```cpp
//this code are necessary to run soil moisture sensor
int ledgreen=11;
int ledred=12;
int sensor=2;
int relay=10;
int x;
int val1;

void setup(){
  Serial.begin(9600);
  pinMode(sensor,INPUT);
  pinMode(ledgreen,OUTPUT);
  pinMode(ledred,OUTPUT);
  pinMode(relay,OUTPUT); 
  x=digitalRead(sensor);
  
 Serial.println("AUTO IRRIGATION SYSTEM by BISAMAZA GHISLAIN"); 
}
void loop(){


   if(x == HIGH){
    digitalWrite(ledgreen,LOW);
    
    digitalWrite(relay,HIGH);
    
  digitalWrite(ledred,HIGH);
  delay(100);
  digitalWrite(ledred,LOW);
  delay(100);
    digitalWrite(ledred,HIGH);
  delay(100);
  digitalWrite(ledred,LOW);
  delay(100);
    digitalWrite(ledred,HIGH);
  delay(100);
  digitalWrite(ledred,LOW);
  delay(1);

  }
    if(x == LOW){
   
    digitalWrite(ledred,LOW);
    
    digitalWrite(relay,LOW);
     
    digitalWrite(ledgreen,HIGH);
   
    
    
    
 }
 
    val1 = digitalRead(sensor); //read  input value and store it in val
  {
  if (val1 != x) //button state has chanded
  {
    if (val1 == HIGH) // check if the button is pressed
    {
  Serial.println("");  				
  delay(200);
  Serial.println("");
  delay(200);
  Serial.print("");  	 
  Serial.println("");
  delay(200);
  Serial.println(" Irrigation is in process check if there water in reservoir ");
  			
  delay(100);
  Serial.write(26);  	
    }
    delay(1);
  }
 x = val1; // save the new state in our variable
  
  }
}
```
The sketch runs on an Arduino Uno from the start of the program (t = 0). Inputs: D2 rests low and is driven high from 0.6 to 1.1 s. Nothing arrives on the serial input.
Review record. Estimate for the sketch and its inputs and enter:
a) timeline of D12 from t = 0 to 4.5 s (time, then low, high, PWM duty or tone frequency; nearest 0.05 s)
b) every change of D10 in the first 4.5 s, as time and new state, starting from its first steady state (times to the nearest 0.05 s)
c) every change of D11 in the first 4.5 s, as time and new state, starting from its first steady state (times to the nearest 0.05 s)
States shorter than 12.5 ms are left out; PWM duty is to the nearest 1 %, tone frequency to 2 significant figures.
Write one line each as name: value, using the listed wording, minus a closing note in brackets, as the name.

timeline of D12 from t = 0 to 4.5 s: 0 s low; 1.3 s high; 1.4 s low; 1.5 s high; 1.6 s low; 1.7 s high; 1.8 s low
every change of D10 in the first 4.5 s, as time and new state, starting from its first steady state: 0 s low; 1.3 s high; 1.8 s low
every change of D11 in the first 4.5 s, as time and new state, starting from its first steady state: 0 s high; 1.3 s low; 1.8 s high
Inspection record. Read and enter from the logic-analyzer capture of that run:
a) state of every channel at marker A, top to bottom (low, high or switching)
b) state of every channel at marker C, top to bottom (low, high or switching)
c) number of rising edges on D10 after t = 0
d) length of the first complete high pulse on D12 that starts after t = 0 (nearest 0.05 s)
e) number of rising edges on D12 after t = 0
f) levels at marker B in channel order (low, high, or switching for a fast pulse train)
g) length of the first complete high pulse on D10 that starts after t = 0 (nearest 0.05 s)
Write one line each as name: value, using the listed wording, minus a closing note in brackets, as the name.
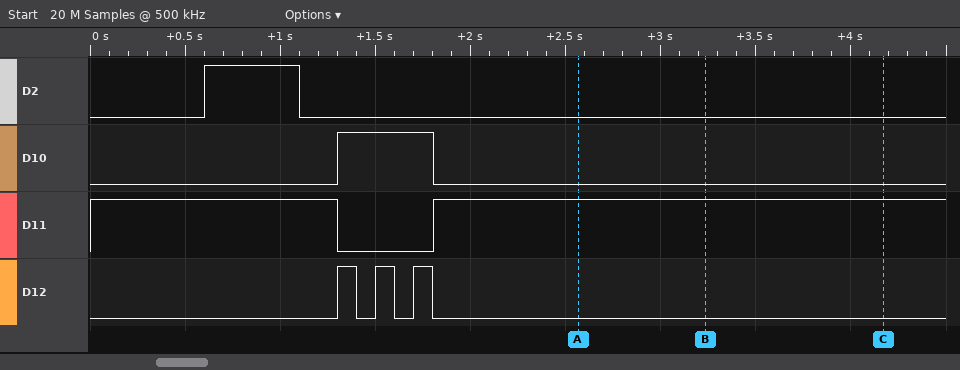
state of every channel at marker A, top to bottom: D2 low, D10 low, D11 high, D12 low
state of every channel at marker C, top to bottom: D2 low, D10 low, D11 high, D12 low
number of rising edges on D10 after t = 0: 1
length of the first complete high pulse on D12 that starts after t = 0: 0.10 s
number of rising edges on D12 after t = 0: 3
levels at marker B in channel order: D2 low, D10 low, D11 high, D12 low
length of the first complete high pulse on D10 that starts after t = 0: 0.50 s
